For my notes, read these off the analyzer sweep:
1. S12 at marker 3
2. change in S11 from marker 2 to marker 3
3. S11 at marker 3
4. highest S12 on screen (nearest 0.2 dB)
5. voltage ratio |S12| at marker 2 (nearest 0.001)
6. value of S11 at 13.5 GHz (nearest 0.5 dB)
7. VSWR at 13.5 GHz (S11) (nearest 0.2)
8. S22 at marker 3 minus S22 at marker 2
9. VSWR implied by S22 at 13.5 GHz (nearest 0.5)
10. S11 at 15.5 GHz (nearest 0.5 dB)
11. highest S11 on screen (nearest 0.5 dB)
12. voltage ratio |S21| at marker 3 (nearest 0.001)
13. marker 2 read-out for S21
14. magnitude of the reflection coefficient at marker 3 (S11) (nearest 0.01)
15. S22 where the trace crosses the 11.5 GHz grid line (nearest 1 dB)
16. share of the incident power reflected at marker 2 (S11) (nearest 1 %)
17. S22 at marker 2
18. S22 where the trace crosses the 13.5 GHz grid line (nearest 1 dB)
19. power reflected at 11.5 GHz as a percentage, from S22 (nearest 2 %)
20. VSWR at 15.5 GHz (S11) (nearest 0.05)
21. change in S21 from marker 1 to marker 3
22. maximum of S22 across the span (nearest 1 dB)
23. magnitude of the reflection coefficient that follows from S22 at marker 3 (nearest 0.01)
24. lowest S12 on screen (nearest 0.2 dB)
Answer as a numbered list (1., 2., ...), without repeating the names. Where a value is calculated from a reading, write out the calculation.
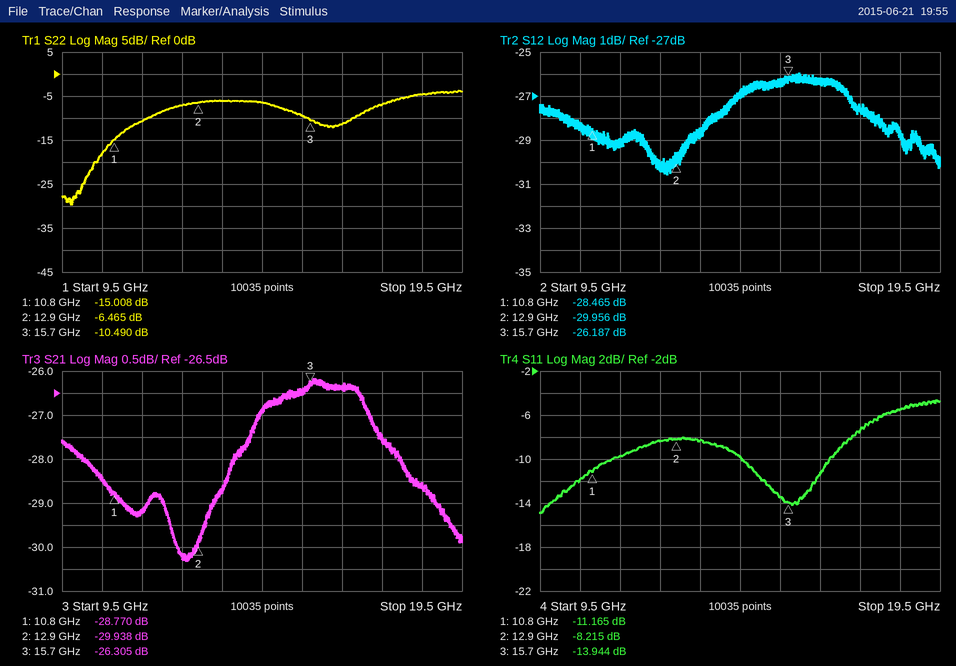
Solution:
1. -26.187 dB
2. -13.944 − (-8.215) = -5.729 dB
3. -13.944 dB
4. -26.0 dB
5. 10^(-29.956/20) ≈ 0.032
6. -8.5 dB
7. |Γ| = 10^(-8.5/20) = 0.3758; VSWR = (1 + 0.3758)/(1 − 0.3758) ≈ 2.2
8. -10.49 − (-6.465) = -4.025 dB
9. |Γ| = 10^(-6/20) = 0.5012; VSWR = (1 + 0.5012)/(1 − 0.5012) ≈ 3.0
10. -13.5 dB
11. -4.5 dB
12. 10^(-26.305/20) ≈ 0.048
13. -29.938 dB
14. 10^(-13.944/20) ≈ 0.20
15. -11 dB
16. 10^(-8.215/10) ≈ 15 %
17. -6.465 dB
18. -6 dB
19. 10^(-11/10) ≈ 8 %
20. |Γ| = 10^(-13.5/20) = 0.2113; VSWR = (1 + 0.2113)/(1 − 0.2113) ≈ 1.54, so 1.55 to the nearest 0.05
21. -26.305 − (-28.77) = 2.465 dB
22. -4 dB
23. 10^(-10.49/20) ≈ 0.30
24. -30.6 dB
